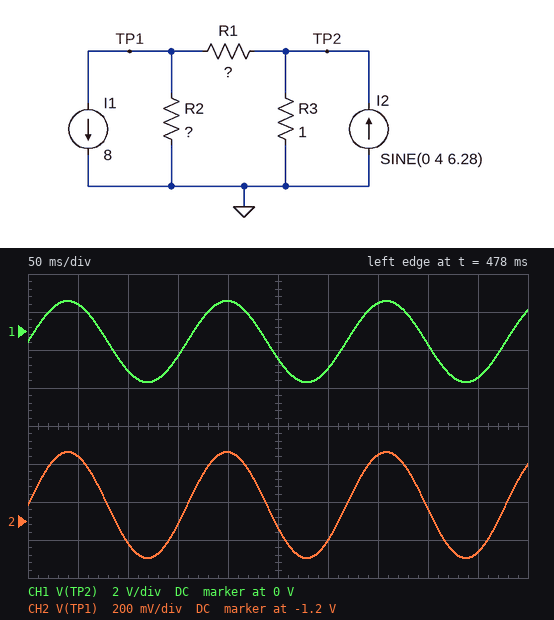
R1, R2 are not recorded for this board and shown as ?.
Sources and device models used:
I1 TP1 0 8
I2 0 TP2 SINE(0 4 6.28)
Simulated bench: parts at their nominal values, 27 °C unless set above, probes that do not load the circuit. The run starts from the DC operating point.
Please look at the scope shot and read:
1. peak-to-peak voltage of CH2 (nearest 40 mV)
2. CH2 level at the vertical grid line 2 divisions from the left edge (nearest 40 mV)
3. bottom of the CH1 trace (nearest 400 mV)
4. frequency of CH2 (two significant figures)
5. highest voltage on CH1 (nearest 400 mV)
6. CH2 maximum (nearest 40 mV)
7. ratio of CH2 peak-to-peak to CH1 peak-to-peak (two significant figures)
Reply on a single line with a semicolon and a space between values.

560 mV; -1.32 V; -2.8 V; 6.3 Hz; 1.6 V; -840 mV; 0.13
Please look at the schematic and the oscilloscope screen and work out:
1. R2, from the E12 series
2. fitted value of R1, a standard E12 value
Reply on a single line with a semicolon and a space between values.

0.15 Ω; 1 Ω
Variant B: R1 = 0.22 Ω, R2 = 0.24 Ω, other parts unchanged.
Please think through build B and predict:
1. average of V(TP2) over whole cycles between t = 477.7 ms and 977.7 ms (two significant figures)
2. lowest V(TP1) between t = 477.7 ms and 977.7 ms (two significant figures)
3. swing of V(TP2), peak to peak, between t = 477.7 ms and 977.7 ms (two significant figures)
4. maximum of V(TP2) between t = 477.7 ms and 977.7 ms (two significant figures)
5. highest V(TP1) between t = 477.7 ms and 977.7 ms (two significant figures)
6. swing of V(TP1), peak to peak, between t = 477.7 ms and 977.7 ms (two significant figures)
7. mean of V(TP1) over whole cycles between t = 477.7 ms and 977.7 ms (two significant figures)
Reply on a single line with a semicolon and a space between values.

-1.3 V; -2.3 V; 2.5 V; -55 mV; -950 mV; 1.3 V; -1.6 V
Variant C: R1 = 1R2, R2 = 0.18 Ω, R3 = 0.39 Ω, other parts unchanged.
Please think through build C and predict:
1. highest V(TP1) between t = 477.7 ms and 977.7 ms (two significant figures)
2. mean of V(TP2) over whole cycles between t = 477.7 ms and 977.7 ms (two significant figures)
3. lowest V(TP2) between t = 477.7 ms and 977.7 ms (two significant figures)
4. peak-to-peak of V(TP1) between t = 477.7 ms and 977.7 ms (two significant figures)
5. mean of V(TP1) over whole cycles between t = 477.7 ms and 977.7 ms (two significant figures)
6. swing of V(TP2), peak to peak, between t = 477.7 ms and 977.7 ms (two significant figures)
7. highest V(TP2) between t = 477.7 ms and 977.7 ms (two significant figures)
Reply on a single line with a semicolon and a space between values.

-1.1 V; -320 mV; -1.5 V; 320 mV; -1.3 V; 2.4 V; 900 mV
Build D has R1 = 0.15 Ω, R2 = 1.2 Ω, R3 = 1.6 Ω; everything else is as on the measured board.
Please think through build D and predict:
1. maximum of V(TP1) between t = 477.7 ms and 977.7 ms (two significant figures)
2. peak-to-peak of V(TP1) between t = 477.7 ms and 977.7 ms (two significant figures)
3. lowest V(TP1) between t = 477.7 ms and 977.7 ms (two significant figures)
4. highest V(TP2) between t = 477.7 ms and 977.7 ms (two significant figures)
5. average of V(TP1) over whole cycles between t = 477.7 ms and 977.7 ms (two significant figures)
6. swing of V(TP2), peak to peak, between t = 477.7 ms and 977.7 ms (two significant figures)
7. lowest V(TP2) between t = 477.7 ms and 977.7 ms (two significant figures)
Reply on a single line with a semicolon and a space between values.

-3.1 V; 5.2 V; -8.3 V; -2.3 V; -5.7 V; 5.9 V; -8.1 V
